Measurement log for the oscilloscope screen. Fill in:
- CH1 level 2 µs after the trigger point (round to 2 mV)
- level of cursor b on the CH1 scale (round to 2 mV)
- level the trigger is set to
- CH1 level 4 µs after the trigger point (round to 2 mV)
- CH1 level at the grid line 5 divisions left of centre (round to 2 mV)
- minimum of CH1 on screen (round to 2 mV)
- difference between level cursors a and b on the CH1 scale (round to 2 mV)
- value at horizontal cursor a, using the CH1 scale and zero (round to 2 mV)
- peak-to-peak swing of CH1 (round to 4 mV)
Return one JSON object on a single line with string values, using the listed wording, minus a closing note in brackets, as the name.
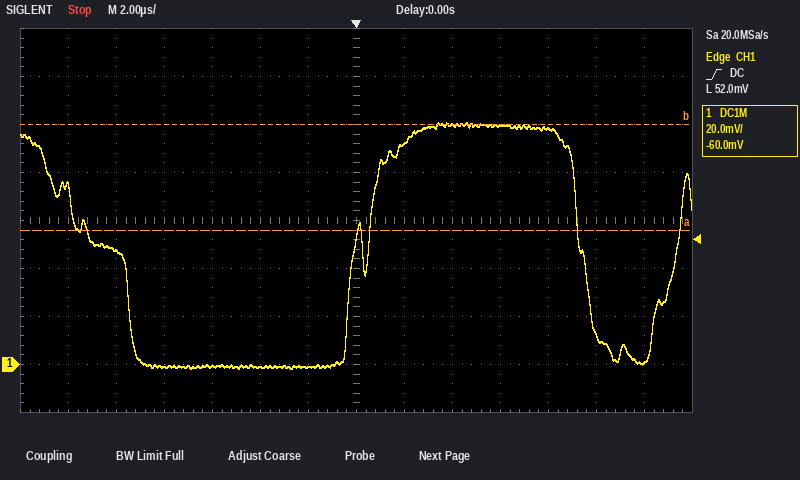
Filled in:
{"CH1 level 2 µs after the trigger point": "92 mV", "level of cursor b on the CH1 scale": "100 mV", "level the trigger is set to": "52.0 mV", "CH1 level 4 µs after the trigger point": "100 mV", "CH1 level at the grid line 5 divisions left of centre": "48 mV", "minimum of CH1 on screen": "-2 mV", "difference between level cursors a and b on the CH1 scale": "44 mV", "value at horizontal cursor a, using the CH1 scale and zero": "56 mV", "peak-to-peak swing of CH1": "104 mV"}
